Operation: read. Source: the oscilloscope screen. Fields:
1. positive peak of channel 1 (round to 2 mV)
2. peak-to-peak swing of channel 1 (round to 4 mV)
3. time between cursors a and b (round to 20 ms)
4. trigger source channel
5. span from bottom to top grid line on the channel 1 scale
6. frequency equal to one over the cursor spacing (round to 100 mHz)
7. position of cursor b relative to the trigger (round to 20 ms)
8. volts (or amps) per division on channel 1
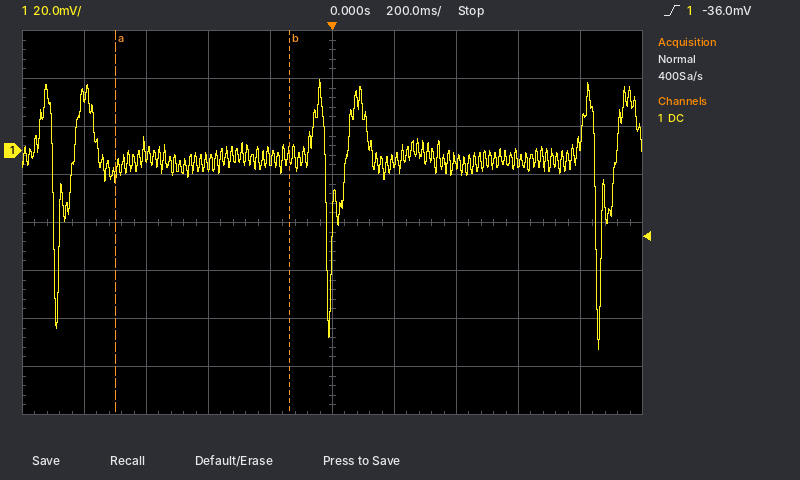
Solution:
30 mV
112 mV
560 ms
channel 1
160 mV
1.8 Hz
-140 ms
20 mV
